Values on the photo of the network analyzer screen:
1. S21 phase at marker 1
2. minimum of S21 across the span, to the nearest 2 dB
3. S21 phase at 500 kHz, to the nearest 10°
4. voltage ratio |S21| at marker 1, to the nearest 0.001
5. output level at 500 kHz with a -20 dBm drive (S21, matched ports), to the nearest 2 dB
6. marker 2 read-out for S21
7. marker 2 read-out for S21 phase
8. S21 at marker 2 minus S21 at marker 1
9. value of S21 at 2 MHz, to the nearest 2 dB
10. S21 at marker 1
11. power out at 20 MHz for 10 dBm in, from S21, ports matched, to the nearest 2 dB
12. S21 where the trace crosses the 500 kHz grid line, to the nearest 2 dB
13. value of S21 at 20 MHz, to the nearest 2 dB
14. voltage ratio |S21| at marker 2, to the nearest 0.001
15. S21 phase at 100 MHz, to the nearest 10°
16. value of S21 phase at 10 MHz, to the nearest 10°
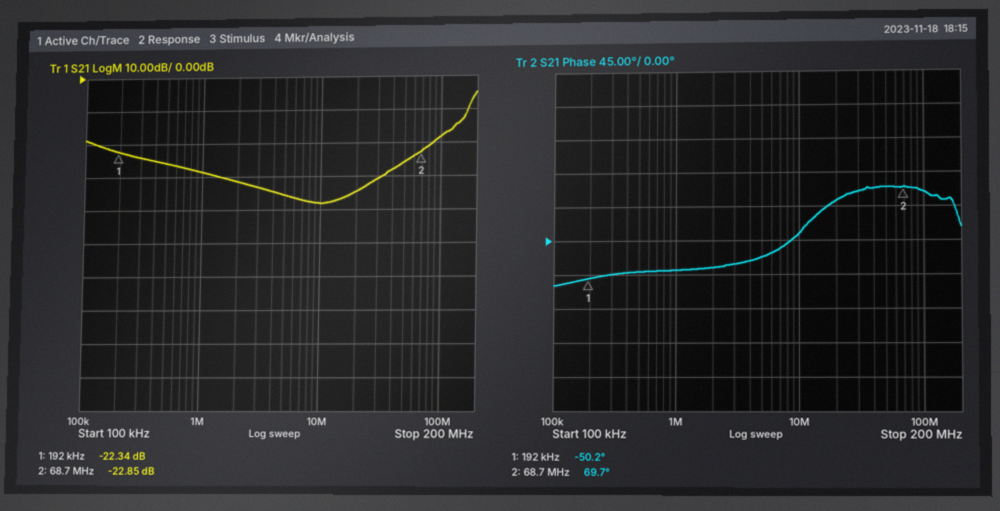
-50.2°
-38 dB
-40°
0.076
-46 dBm
-22.85 dB
69.7°
-0.51 dB
-32 dB
-22.34 dB
-24 dBm
-26 dB
-34 dB
0.072
60°
10°
